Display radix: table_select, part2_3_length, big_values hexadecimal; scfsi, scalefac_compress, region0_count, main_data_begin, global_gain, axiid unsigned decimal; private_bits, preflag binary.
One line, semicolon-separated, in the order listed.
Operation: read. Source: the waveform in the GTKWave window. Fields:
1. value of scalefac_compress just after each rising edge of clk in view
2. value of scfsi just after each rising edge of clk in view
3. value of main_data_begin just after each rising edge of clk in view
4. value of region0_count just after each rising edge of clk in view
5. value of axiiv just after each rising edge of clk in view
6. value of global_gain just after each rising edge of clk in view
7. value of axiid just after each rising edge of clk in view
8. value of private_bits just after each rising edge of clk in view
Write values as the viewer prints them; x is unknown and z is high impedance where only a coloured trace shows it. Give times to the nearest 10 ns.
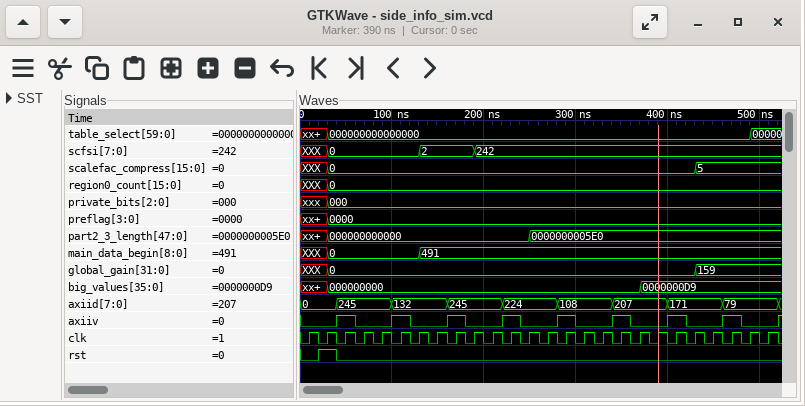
XXX, 0, 0, 0, 0, 0, 0, 0, 0, 0, 0, 0, 0, 0, 0, 0, 0, 0, 0, 0, 0, 5, 5, 5, 5, 5; XXX, 0, 0, 0, 0, 0, 2, 2, 2, 242, 242, 242, 242, 242, 242, 242, 242, 242, 242, 242, 242, 242, 242, 242, 242, 242; XXX, 0, 0, 0, 0, 0, 491, 491, 491, 491, 491, 491, 491, 491, 491, 491, 491, 491, 491, 491, 491, 491, 491, 491, 491, 491; XXX, 0, 0, 0, 0, 0, 0, 0, 0, 0, 0, 0, 0, 0, 0, 0, 0, 0, 0, 0, 0, 0, 0, 0, 0, 0; 0 0 1 0 0 1 0 0 1 0 0 1 0 0 1 0 0 1 0 0 1 0 0 1 0 0; XXX, 0, 0, 0, 0, 0, 0, 0, 0, 0, 0, 0, 0, 0, 0, 0, 0, 0, 0, 0, 0, 159, 159, 159, 159, 159; 0, 0, 245, 245, 245, 132, 132, 132, 245, 245, 245, 224, 224, 224, 108, 108, 108, 207, 207, 207, 171, 171, 171, 79, 79, 79; xxx, 000, 000, 000, 000, 000, 000, 000, 000, 000, 000, 000, 000, 000, 000, 000, 000, 000, 000, 000, 000, 000, 000, 000, 000, 000
